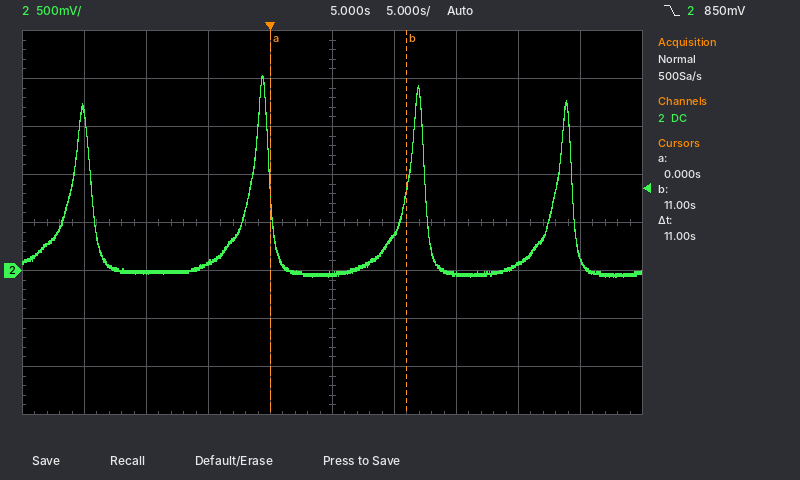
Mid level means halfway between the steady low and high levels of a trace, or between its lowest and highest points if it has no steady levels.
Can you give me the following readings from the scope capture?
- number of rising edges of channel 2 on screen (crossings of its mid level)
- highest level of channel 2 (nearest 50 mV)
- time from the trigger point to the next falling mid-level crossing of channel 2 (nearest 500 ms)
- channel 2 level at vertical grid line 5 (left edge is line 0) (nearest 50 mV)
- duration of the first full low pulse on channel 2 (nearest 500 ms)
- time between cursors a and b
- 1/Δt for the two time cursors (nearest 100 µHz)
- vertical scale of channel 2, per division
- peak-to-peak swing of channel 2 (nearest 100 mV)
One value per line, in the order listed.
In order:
4
2.05 V
12.5 s
-50 mV
13.0 s
11 s
90.9 mHz
500 mV
2.10 V
